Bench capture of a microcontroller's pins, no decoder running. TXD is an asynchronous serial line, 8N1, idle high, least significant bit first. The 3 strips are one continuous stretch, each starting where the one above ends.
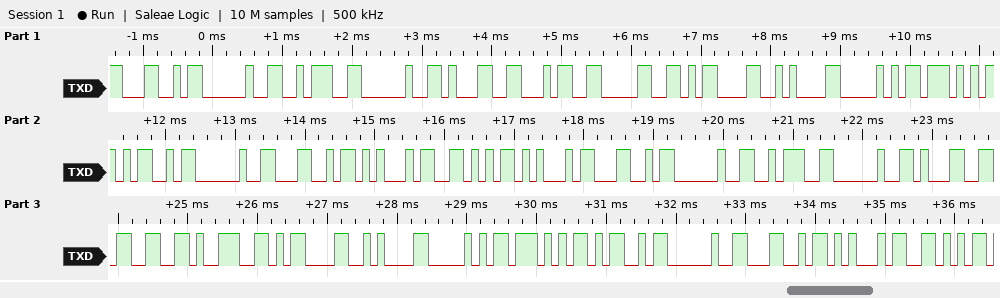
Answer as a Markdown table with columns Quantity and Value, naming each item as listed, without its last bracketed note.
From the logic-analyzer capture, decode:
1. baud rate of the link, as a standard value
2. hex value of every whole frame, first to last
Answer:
| Quantity | Value |
|---|---|
| baud rate of the link, as a standard value | 9600 baud |
| hex value of every whole frame, first to last | 4C 20 3A 20 31 34 30 0D 0A 50 57 4D 20 4C 45 56 45 4C 20 3A 20 31 33 39 0D 0A 50 57 4D 20 4C 45 56 |
